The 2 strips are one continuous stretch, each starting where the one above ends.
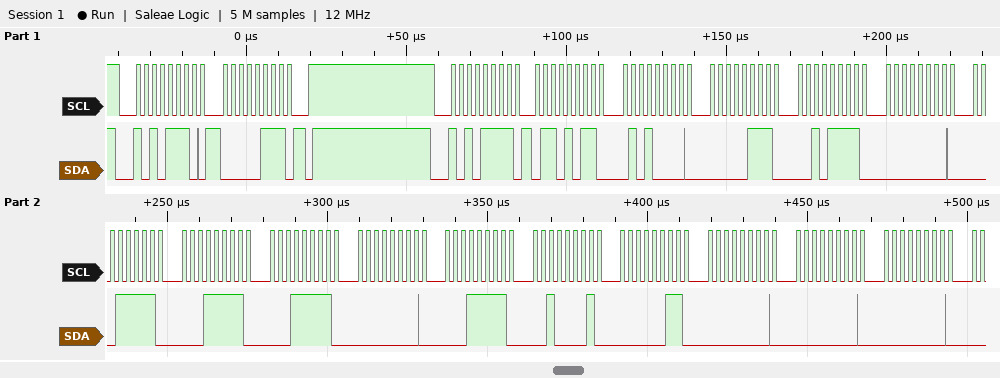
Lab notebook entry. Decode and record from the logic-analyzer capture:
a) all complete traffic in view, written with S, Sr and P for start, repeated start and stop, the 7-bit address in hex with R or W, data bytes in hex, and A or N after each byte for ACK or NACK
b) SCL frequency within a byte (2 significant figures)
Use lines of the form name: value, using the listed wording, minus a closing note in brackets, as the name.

all complete traffic in view, written with S, Sr and P for start, repeated start and stop, the 7-bit address in hex with R or W, data bytes in hex, and A or N after each byte for ACK or NACK: S 57W A 07 A P S 57R A 6B A 50 A 07 A 2F A 00 A 1F A 1F A 1F A 00 A 1F A 21 A 03 A 00 A 00 A 00 A
SCL frequency within a byte: 400 kHz
